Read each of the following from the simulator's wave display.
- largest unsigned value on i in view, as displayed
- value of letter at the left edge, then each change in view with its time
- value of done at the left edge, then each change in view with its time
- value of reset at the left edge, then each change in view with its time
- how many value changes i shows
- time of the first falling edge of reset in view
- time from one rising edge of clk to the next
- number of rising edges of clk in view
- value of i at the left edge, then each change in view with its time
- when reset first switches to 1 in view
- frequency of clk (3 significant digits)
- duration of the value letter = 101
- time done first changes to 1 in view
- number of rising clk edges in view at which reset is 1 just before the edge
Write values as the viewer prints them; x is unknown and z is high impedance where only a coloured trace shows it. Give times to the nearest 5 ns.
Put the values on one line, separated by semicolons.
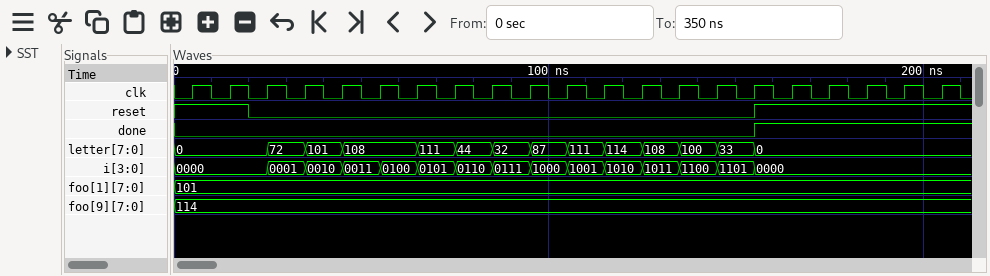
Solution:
1101; 0, 72 at 25 ns, 101 at 35 ns, 108 at 45 ns, 111 at 65 ns, 44 at 75 ns, 32 at 85 ns, 87 at 95 ns, 111 at 105 ns, 114 at 115 ns, 108 at 125 ns, 100 at 135 ns, 33 at 145 ns, 0 at 155 ns; 0, 1 at 155 ns; 1, 0 at 20 ns, 1 at 155 ns; 14; 20 ns; 10 ns; 21; 0000, 0001 at 25 ns, 0010 at 35 ns, 0011 at 45 ns, 0100 at 55 ns, 0101 at 65 ns, 0110 at 75 ns, 0111 at 85 ns, 1000 at 95 ns, 1001 at 105 ns, 1010 at 115 ns, 1011 at 125 ns, 1100 at 135 ns, 1101 at 145 ns, 0000 at 155 ns; 155 ns; 100 MHz; 10 ns; 155 ns; 7
